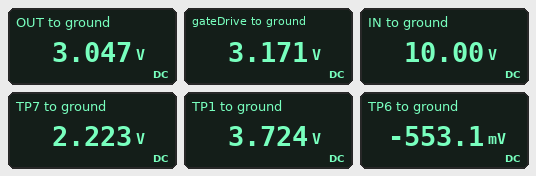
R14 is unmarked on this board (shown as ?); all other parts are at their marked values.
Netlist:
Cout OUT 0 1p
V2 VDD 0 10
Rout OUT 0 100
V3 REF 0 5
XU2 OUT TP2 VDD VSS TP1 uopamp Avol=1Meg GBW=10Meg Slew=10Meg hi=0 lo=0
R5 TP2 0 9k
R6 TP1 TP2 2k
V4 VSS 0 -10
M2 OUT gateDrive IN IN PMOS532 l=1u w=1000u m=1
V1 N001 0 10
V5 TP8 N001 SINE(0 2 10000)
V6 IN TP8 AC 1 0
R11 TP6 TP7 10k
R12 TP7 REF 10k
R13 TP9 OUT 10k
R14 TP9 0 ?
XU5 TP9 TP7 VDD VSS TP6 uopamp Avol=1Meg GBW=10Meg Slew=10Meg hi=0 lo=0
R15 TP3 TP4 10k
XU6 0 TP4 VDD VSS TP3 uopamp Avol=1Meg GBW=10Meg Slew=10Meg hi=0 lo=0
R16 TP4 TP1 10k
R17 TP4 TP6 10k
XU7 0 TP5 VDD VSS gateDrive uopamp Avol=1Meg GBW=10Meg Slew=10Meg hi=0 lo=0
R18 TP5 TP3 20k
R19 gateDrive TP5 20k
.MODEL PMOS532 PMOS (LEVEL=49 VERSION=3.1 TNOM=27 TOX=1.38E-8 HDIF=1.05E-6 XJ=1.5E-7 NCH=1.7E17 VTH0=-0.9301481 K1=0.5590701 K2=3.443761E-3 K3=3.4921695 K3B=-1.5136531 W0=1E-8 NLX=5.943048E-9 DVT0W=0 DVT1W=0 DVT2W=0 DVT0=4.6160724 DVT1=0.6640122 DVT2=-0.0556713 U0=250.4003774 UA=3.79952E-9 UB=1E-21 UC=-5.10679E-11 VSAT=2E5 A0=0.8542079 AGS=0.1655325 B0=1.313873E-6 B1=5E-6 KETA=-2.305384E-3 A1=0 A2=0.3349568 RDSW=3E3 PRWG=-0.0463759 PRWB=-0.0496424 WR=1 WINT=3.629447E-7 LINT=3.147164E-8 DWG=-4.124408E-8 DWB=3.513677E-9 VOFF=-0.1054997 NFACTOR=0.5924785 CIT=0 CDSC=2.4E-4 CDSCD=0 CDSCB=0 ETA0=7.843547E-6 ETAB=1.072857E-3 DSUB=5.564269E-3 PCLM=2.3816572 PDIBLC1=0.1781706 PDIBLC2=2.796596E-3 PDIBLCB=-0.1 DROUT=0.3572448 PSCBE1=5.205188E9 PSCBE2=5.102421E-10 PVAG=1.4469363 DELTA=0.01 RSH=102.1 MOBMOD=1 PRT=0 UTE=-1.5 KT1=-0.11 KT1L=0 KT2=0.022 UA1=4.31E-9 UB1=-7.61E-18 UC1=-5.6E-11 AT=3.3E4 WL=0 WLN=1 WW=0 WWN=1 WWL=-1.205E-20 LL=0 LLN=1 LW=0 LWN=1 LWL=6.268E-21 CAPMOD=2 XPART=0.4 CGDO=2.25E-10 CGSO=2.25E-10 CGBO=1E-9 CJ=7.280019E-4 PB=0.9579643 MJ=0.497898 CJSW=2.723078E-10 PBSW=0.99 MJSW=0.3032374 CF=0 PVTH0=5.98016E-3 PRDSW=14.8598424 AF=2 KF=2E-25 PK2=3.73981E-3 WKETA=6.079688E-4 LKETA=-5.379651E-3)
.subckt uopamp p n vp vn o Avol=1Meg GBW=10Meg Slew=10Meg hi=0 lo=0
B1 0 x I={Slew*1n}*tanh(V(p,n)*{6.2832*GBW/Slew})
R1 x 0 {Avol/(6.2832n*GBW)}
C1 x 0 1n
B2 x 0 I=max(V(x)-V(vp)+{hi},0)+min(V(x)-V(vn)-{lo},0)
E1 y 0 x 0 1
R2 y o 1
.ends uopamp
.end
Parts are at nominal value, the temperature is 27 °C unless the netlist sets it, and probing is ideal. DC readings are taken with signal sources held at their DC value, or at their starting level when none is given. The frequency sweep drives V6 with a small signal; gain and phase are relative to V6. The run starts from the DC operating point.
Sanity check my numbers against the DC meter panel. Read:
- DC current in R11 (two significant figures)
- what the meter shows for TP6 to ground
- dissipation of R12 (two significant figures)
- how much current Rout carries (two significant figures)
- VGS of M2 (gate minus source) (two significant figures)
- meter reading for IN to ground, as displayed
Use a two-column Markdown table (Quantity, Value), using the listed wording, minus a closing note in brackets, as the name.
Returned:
| Quantity | Value |
|---|---|
| DC current in R11 | 280 µA |
| what the meter shows for TP6 to ground | -553.1 mV |
| dissipation of R12 | 770 µW |
| how much current Rout carries | 30 mA |
| VGS of M2 (gate minus source) | -6.8 V |
| meter reading for IN to ground, as displayed | 10.00 V |
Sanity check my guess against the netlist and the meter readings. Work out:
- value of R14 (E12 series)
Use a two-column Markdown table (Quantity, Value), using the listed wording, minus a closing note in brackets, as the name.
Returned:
| Quantity | Value |
|---|---|
| value of R14 | 27 kΩ |
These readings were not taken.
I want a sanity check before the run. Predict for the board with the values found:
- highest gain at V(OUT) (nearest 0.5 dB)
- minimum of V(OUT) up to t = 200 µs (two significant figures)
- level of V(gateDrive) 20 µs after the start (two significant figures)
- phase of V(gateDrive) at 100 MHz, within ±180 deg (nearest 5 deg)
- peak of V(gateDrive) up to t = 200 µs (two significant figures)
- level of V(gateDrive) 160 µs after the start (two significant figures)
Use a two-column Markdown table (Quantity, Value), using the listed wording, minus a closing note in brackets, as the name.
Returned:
| Quantity | Value |
|---|---|
| highest gain at V(OUT) | -8.5 dB |
| minimum of V(OUT) up to t = 200 µs | 2.5 V |
| level of V(gateDrive) 20 µs after the start | 4.6 V |
| phase of V(gateDrive) at 100 MHz, within ±180 deg | 90 deg |
| peak of V(gateDrive) up to t = 200 µs | 4.7 V |
| level of V(gateDrive) 160 µs after the start | 2.3 V |
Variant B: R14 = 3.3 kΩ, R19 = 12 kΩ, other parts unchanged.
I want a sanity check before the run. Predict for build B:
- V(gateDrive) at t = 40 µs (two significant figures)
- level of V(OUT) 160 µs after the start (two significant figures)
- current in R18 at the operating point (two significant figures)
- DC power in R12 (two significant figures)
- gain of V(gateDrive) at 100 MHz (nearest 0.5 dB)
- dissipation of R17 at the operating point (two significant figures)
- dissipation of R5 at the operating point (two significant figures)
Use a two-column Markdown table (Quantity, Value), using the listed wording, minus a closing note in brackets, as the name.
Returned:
| Quantity | Value |
|---|---|
| V(gateDrive) at t = 40 µs | 630 mV |
| level of V(OUT) 160 µs after the start | 2.8 V |
| current in R18 at the operating point | 20 µA |
| DC power in R12 | 1.8 mW |
| gain of V(gateDrive) at 100 MHz | -58.5 dB |
| dissipation of R17 at the operating point | 1.2 mW |
| dissipation of R5 at the operating point | 1.1 mW |
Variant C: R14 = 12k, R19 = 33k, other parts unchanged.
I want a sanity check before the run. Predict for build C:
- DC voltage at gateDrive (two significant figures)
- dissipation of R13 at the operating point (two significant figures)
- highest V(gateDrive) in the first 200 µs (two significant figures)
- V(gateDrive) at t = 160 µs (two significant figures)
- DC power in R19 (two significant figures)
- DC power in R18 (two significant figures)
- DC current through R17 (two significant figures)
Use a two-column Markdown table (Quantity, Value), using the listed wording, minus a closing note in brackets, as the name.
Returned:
| Quantity | Value |
|---|---|
| DC voltage at gateDrive | 3.3 V |
| dissipation of R13 at the operating point | 190 µW |
| highest V(gateDrive) in the first 200 µs | 5.1 V |
| V(gateDrive) at t = 160 µs | 2.1 V |
| DC power in R19 | 330 µW |
| DC power in R18 | 200 µW |
| DC current through R17 | 170 µA |
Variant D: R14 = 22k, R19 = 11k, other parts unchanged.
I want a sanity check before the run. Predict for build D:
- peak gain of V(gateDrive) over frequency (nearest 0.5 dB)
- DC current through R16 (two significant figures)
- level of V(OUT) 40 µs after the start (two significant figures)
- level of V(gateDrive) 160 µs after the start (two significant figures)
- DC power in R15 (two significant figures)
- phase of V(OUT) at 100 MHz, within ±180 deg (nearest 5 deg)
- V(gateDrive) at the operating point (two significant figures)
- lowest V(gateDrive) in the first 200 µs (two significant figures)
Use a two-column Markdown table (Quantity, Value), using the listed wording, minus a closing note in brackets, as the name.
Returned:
| Quantity | Value |
|---|---|
| peak gain of V(gateDrive) over frequency | -7.0 dB |
| DC current through R16 | 380 µA |
| level of V(OUT) 40 µs after the start | 3.5 V |
| level of V(gateDrive) 160 µs after the start | 1.2 V |
| DC power in R15 | 960 µW |
| phase of V(OUT) at 100 MHz, within ±180 deg | -5 deg |
| V(gateDrive) at the operating point | 1.7 V |
| lowest V(gateDrive) in the first 200 µs | 810 mV |
